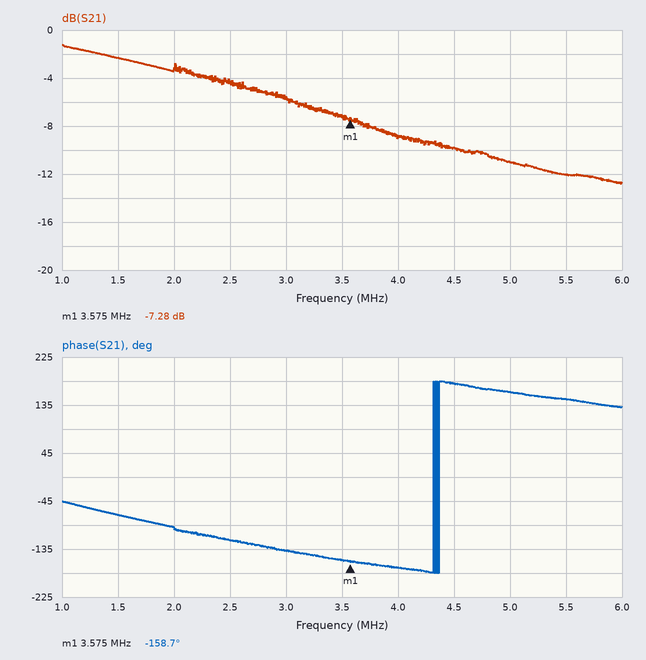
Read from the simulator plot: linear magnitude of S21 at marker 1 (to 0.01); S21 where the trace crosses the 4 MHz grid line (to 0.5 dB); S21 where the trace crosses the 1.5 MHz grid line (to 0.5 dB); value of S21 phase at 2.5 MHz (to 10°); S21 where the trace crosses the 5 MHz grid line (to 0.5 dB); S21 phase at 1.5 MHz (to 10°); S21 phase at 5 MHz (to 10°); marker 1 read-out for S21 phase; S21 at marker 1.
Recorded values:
0.43
-9.0 dB
-2.5 dB
-120°
-11.0 dB
-70°
160°
-158.7°
-7.28 dB
